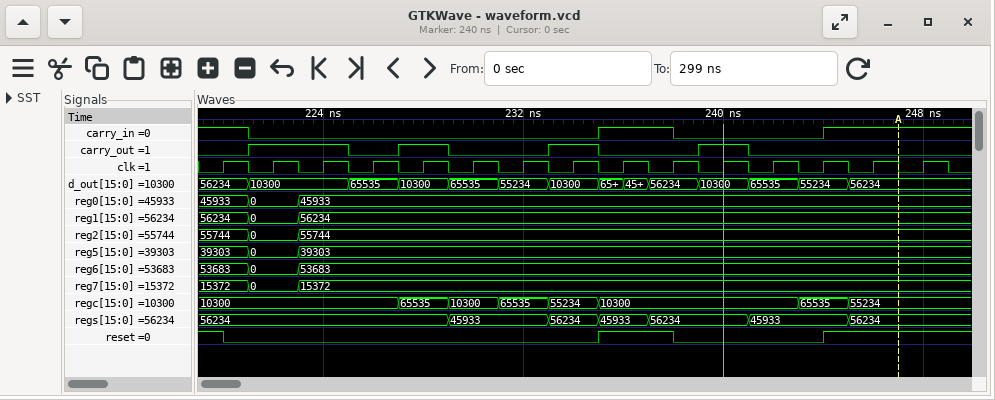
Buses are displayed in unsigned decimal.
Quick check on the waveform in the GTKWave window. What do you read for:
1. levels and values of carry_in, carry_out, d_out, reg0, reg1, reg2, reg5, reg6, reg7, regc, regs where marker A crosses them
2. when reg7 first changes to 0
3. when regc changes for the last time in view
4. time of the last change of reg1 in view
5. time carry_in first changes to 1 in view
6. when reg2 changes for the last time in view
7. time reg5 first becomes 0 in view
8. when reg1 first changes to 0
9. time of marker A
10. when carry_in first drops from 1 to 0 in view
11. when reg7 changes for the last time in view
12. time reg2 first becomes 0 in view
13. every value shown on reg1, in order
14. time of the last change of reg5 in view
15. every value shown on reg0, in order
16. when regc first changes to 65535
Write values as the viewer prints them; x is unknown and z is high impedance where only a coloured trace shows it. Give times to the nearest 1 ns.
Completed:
carry_in=1, carry_out=0, d_out=56234, reg0=45933, reg1=56234, reg2=55744, reg5=39303, reg6=53683, reg7=15372, regc=55234, regs=56234
221 ns
245 ns
223 ns
235 ns
223 ns
221 ns
221 ns
247 ns
221 ns
223 ns
221 ns
56234, 0, 56234
223 ns
45933, 0, 45933
227 ns
